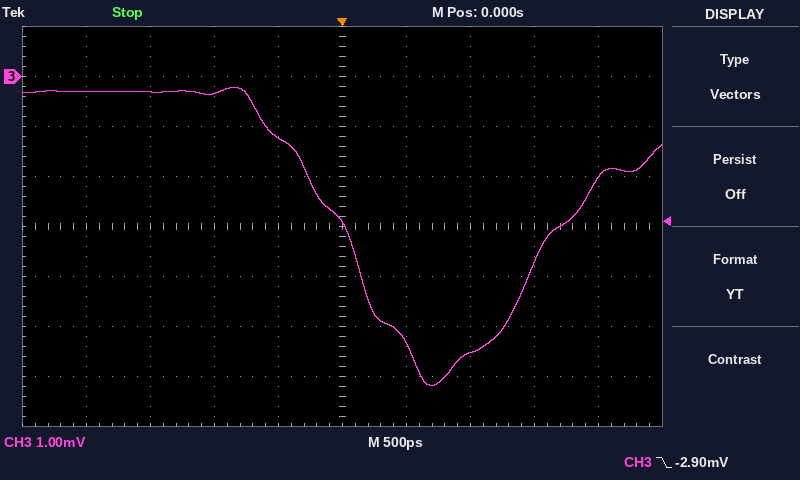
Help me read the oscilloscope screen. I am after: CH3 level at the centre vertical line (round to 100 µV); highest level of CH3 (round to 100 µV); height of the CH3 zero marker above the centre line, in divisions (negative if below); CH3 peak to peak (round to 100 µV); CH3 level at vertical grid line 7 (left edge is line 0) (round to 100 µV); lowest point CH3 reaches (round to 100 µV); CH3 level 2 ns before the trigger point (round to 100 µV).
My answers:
-2.9 mV
-200 µV
+3.0 div
6.0 mV
-5.5 mV
-6.2 mV
-300 µV
